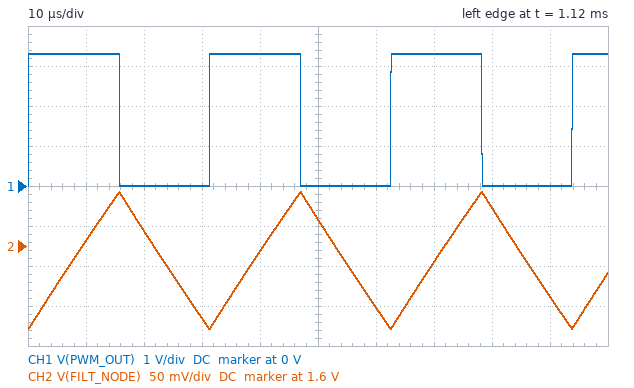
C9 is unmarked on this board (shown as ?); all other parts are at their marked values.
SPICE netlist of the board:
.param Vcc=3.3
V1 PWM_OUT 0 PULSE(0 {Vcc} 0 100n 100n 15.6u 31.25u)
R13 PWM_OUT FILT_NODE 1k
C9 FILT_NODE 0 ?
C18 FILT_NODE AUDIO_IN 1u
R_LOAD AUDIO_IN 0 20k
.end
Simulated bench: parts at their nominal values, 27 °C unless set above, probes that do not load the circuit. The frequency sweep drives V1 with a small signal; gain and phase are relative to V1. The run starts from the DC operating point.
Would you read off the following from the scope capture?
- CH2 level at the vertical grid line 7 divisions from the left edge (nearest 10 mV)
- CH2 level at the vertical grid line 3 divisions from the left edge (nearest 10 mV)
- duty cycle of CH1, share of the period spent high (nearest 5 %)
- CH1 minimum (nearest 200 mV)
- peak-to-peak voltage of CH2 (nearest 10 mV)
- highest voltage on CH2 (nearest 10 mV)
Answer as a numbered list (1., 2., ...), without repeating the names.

1. 1.58 V
2. 1.51 V
3. 50 %
4. 0 V
5. 170 mV
6. 1.67 V
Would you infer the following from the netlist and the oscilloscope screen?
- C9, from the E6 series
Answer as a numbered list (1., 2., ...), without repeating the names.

1. 150 nF
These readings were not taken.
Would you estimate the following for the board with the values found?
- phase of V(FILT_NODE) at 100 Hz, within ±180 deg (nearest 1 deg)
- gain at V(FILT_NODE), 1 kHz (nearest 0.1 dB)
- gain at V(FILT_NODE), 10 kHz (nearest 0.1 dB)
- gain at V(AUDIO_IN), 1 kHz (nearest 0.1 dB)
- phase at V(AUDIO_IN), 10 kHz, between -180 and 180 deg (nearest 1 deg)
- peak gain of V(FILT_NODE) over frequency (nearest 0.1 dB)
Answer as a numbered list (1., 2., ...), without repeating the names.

1. -5 deg
2. -3.0 dB
3. -19.5 dB
4. -3.0 dB
5. -84 deg
6. 0 dB
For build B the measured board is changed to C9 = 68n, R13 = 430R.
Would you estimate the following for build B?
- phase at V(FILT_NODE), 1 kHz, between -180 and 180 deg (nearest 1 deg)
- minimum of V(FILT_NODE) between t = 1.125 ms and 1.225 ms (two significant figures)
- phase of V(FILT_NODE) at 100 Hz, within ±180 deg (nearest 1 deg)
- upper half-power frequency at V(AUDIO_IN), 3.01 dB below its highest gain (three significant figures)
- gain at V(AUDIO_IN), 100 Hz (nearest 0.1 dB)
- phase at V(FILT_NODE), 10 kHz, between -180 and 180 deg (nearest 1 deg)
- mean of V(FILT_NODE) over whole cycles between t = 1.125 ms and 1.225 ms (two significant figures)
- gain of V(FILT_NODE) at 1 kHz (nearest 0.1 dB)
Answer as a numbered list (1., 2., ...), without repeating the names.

1. -10 deg
2. 1.2 V
3. -1 deg
4. 5.58 kHz
5. -0.2 dB
6. -61 deg
7. 1.6 V
8. -0.3 dB
